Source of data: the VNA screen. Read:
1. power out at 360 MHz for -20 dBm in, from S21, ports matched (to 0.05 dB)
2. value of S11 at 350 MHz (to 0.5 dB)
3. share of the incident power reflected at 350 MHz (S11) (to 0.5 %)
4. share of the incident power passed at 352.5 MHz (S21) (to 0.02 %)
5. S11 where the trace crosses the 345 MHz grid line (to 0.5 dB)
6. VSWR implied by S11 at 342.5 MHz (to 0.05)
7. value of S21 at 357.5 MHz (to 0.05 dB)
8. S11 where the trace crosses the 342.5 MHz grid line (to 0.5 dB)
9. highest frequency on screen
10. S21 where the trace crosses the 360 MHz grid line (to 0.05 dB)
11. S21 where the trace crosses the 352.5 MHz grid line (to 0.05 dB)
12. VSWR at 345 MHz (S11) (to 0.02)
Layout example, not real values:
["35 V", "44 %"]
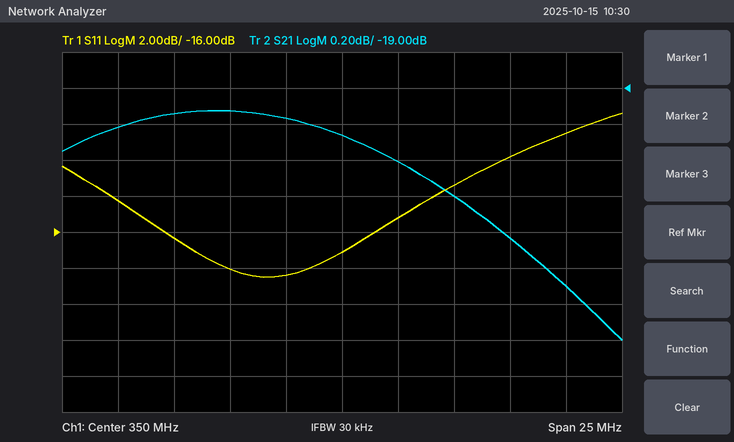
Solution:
["-40.10 dBm", "-17.0 dB", "2.0 %", "1.14 %", "-18.0 dB", "1.35", "-19.85 dB", "-16.5 dB", "362.5 MHz", "-20.10 dB", "-19.40 dB", "1.28"]
